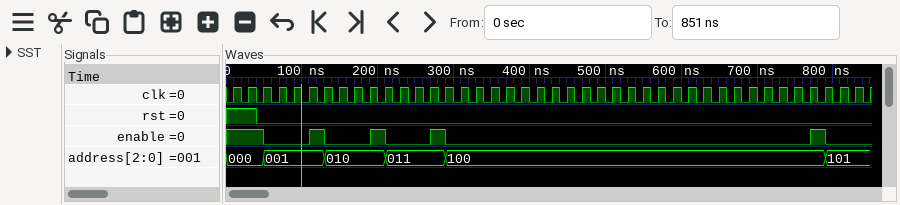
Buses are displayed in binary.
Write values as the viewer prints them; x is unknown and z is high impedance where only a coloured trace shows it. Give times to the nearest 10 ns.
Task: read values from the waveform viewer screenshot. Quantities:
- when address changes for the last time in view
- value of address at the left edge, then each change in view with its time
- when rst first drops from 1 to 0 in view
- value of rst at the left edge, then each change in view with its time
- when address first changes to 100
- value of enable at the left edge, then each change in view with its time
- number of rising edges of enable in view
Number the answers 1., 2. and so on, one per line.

1. 790 ns
2. 000, 001 at 50 ns, 010 at 130 ns, 011 at 210 ns, 100 at 290 ns, 101 at 790 ns
3. 40 ns
4. 1, 0 at 40 ns
5. 290 ns
6. 1, 0 at 50 ns, 1 at 110 ns, 0 at 130 ns, 1 at 190 ns, 0 at 210 ns, 1 at 270 ns, 0 at 290 ns, 1 at 770 ns, 0 at 790 ns
7. 4
